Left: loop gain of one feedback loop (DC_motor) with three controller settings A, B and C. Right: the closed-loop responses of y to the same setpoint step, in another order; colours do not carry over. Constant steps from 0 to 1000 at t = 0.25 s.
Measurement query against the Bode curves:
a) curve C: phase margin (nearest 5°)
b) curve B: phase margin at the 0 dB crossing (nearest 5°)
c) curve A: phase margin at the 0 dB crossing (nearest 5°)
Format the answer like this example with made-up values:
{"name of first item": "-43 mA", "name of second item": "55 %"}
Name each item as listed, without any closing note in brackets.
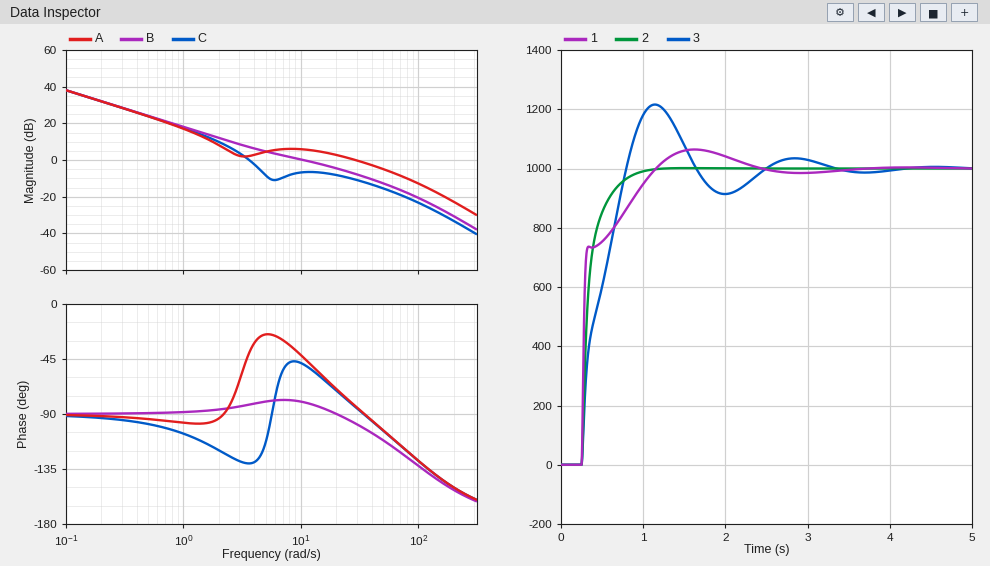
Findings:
{"curve C: phase margin": "50°", "curve B: phase margin at the 0 dB crossing": "100°", "curve A: phase margin at the 0 dB crossing": "95°"}
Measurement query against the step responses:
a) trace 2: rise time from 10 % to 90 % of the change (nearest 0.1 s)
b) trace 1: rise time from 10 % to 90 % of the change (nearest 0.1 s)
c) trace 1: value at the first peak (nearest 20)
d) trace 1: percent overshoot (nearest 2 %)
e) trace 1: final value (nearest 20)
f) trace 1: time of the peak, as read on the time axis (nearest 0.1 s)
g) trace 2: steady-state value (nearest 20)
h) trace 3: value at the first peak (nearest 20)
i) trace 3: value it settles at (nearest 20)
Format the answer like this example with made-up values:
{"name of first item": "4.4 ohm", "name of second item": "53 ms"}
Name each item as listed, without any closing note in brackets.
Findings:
{"trace 2: rise time from 10 % to 90 % of the change": "0.3 s", "trace 1: rise time from 10 % to 90 % of the change": "0.6 s", "trace 1: value at the first peak": "1060", "trace 1: percent overshoot": "6 %", "trace 1: final value": "1000", "trace 1: time of the peak, as read on the time axis": "1.6 s", "trace 2: steady-state value": "1000", "trace 3: value at the first peak": "1220", "trace 3: value it settles at": "1000"}
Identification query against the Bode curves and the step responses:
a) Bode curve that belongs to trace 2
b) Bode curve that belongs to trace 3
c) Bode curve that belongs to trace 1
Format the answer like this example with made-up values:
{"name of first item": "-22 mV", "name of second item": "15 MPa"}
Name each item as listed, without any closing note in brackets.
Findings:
{"Bode curve that belongs to trace 2": "B", "Bode curve that belongs to trace 3": "C", "Bode curve that belongs to trace 1": "A"}
